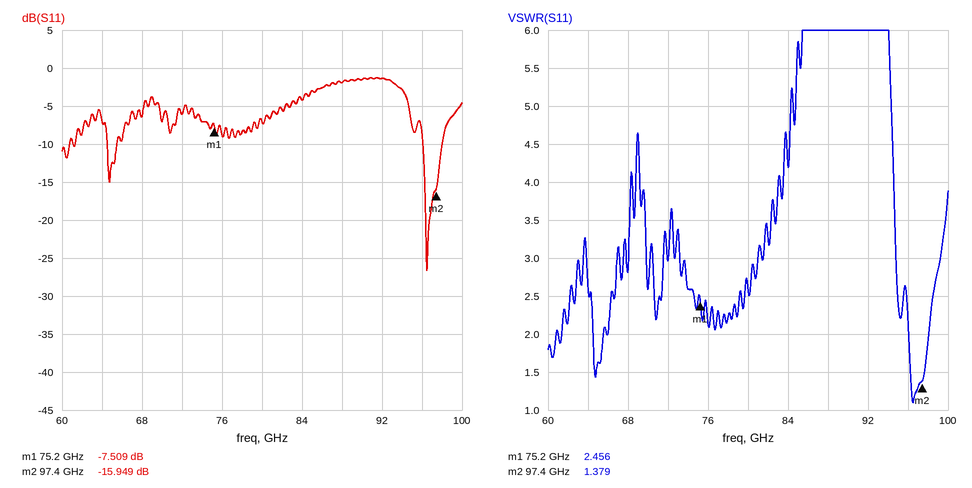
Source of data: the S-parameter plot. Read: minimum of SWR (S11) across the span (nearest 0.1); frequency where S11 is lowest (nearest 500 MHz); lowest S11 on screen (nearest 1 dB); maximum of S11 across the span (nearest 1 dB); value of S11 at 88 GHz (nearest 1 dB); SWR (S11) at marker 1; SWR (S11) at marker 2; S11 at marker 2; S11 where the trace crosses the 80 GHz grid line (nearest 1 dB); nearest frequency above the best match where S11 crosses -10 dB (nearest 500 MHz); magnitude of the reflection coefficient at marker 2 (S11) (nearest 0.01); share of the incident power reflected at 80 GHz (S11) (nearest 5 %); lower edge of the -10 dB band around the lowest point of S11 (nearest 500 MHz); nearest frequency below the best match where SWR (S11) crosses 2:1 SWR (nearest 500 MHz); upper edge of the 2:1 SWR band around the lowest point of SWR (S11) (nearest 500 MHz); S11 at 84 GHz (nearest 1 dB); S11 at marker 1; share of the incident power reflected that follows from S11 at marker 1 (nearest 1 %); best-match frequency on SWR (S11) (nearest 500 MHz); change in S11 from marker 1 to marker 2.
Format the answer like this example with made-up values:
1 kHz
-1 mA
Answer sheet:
1.1
96.5 GHz
-27 dB
-1 dB
-2 dB
2.456
1.379
-15.949 dB
-7 dB
98.0 GHz
0.16
20 %
96.0 GHz
96.0 GHz
98.0 GHz
-4 dB
-7.509 dB
18 %
96.5 GHz
-8.440 dB
